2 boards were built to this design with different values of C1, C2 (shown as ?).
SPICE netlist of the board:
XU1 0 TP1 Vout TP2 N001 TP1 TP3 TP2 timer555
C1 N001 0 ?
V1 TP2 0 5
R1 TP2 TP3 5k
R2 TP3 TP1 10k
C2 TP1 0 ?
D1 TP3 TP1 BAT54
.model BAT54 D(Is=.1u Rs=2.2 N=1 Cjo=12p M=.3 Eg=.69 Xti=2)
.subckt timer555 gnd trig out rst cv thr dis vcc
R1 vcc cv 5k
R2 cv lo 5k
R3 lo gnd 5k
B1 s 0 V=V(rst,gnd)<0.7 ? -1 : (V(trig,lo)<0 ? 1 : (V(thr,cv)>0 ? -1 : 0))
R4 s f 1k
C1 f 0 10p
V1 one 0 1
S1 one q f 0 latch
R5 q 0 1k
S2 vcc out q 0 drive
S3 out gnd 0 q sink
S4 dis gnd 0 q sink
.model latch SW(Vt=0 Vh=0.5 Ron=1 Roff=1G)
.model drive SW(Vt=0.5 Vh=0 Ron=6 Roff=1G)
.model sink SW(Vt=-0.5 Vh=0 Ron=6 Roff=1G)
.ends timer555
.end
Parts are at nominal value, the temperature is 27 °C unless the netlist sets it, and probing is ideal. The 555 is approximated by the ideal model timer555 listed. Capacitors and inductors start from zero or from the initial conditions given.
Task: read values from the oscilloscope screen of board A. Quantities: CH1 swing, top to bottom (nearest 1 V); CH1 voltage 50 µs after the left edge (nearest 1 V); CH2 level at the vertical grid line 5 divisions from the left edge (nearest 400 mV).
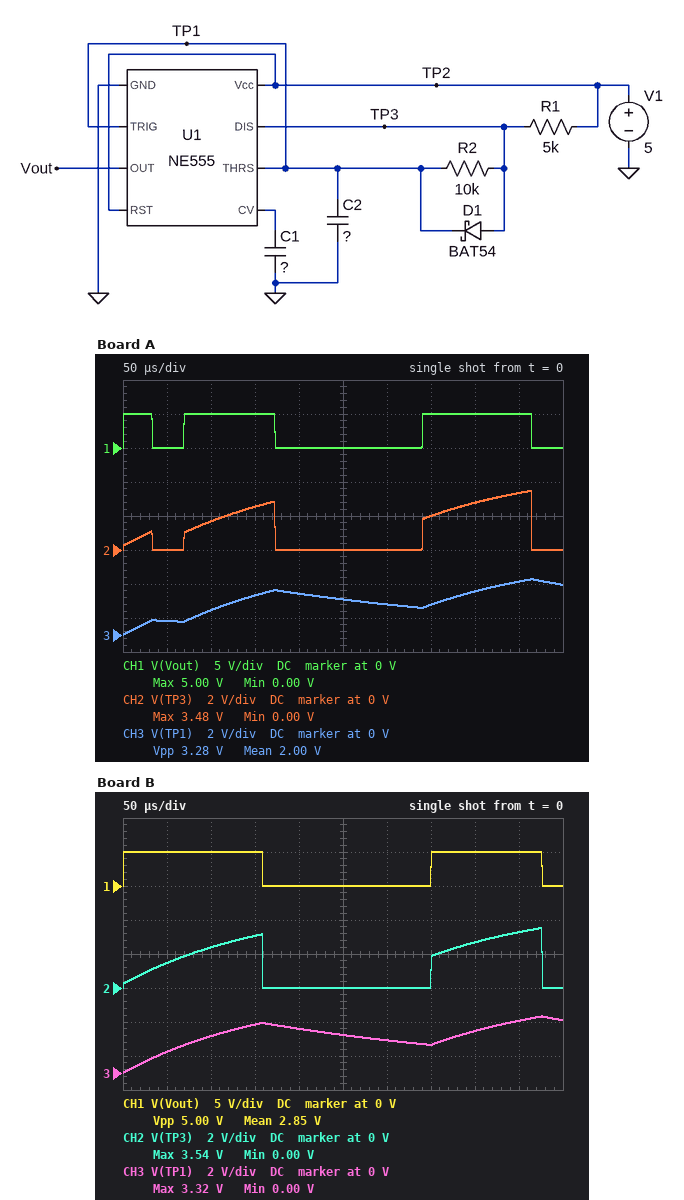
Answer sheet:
5 V
0 V
0 V
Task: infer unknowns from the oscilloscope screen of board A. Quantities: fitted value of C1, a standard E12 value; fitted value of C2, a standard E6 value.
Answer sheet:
33 nF
33 nF
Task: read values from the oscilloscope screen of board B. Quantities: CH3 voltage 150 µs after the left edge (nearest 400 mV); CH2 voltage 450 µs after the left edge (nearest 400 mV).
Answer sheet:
2.8 V
3.2 V
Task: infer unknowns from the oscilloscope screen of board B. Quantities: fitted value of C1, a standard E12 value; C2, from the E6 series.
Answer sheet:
22 nF
33 nF
